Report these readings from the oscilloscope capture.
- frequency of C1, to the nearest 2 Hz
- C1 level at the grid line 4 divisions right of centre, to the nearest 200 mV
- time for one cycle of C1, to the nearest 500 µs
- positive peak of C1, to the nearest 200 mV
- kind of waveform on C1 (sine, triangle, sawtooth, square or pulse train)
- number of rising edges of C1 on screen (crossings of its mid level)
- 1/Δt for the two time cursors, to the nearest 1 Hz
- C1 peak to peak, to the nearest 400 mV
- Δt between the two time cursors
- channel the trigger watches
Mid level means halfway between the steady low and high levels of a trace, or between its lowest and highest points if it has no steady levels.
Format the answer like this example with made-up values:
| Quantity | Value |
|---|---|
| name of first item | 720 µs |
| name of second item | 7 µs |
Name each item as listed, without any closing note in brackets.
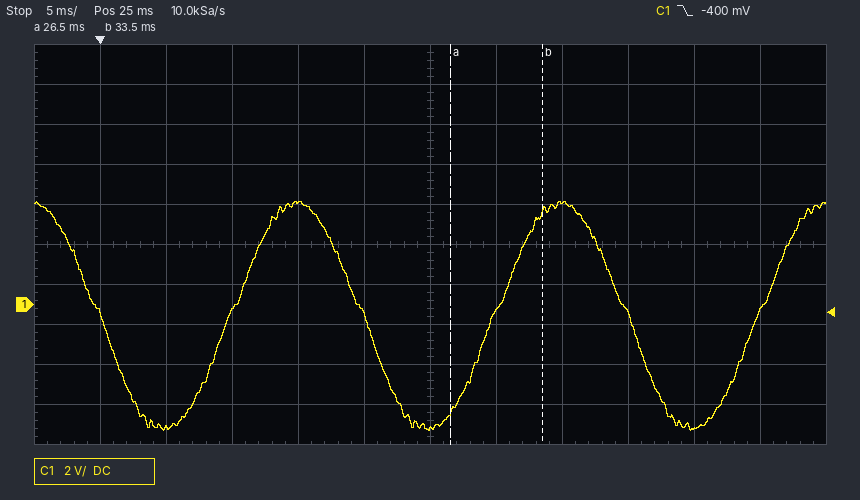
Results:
| Quantity | Value |
|---|---|
| frequency of C1, to the nearest 2 Hz | 50 Hz |
| C1 level at the grid line 4 divisions right of centre, to the nearest 200 mV | -6.2 V |
| time for one cycle of C1, to the nearest 500 µs | 20.0 ms |
| positive peak of C1, to the nearest 200 mV | 5.2 V |
| kind of waveform on C1 | sine |
| number of rising edges of C1 on screen | 3 |
| 1/Δt for the two time cursors, to the nearest 1 Hz | 143 Hz |
| C1 peak to peak, to the nearest 400 mV | 11.6 V |
| Δt between the two time cursors | 7.0 ms |
| channel the trigger watches | C1 |
